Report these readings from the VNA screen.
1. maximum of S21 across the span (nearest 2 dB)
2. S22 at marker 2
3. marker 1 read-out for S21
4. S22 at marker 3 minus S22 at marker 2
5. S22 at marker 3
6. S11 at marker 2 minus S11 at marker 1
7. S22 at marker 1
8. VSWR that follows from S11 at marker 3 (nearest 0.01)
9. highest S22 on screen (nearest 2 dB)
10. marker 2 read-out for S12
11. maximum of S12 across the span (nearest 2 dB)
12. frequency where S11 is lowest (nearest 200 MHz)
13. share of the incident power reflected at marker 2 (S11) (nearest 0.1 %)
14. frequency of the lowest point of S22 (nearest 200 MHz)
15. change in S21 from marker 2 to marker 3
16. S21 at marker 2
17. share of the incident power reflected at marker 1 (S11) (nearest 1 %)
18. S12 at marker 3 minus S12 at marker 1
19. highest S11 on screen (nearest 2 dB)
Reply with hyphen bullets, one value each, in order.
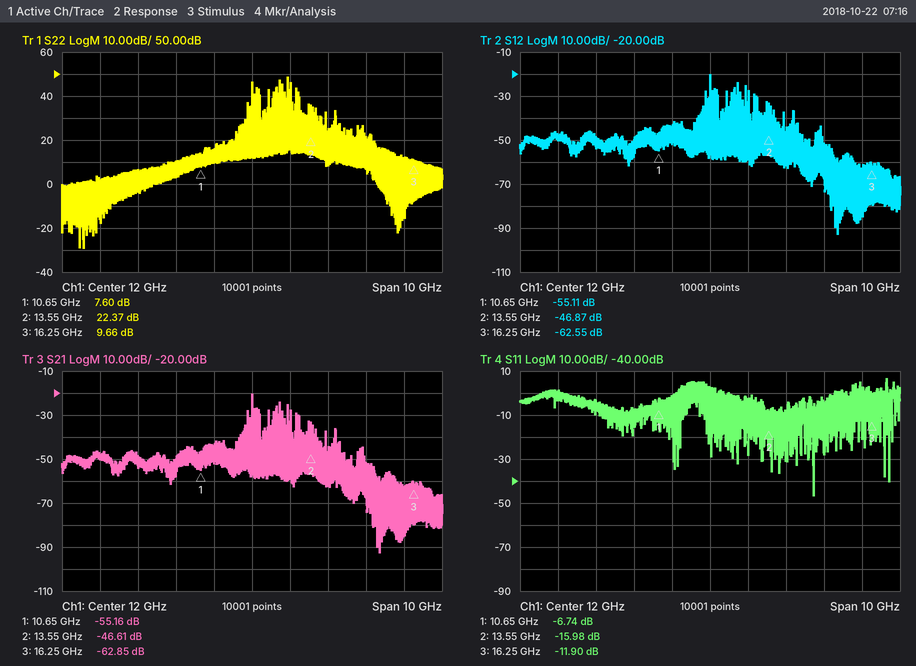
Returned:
- -20 dB
- 22.37 dB
- -55.16 dB
- -12.71 dB
- 9.66 dB
- -9.24 dB
- 7.60 dB
- 1.68
- 48 dB
- -46.87 dB
- -20 dB
- 14.8 GHz
- 2.5 %
- 7.6 GHz
- -16.24 dB
- -46.61 dB
- 21 %
- -7.44 dB
- 6 dB
